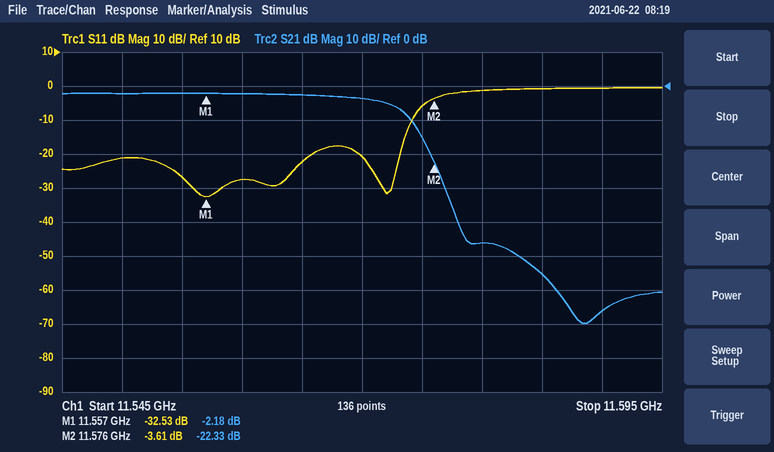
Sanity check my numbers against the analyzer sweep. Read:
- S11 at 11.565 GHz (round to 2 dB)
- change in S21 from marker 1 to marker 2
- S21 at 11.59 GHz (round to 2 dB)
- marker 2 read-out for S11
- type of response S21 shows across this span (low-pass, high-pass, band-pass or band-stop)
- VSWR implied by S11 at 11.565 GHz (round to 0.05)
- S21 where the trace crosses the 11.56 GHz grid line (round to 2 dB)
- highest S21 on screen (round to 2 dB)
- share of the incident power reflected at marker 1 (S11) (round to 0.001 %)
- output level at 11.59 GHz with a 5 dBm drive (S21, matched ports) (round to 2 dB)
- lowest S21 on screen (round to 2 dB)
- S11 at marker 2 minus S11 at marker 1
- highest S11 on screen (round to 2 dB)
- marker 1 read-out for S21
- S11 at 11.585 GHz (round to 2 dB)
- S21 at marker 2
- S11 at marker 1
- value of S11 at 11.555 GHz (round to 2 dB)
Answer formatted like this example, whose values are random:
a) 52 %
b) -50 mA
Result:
a) -22 dB
b) -20.15 dB
c) -66 dB
d) -3.61 dB
e) low-pass
f) 1.15
g) -2 dB
h) -2 dB
i) 0.056 %
j) -62 dBm
k) -70 dB
l) 28.92 dB
m) 0 dB
n) -2.18 dB
o) 0 dB
p) -22.33 dB
q) -32.53 dB
r) -26 dB
